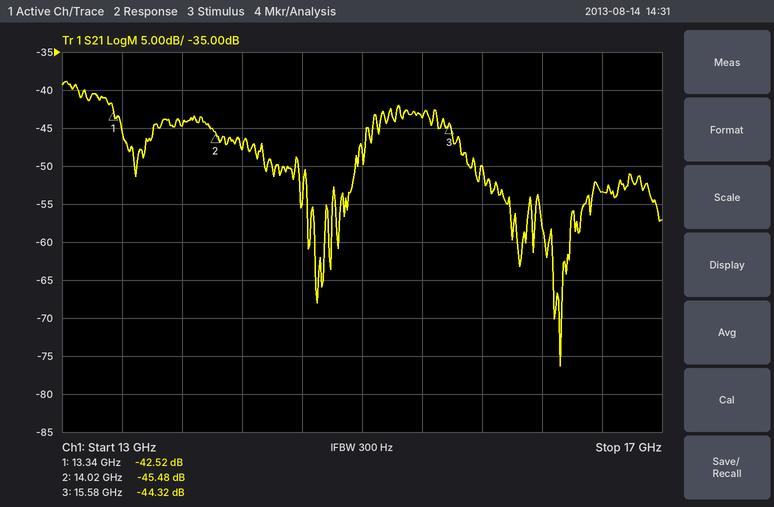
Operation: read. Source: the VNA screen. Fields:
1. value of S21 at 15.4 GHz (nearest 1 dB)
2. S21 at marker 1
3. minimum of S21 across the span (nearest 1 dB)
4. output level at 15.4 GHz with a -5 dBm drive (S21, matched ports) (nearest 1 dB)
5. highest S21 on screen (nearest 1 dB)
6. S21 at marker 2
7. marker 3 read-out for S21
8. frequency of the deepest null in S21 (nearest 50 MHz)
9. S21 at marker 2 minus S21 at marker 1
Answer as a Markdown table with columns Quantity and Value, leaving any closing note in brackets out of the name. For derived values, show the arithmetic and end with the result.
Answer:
| Quantity | Value |
|---|---|
| value of S21 at 15.4 GHz | -44 dB |
| S21 at marker 1 | -42.52 dB |
| minimum of S21 across the span | -76 dB |
| output level at 15.4 GHz with a -5 dBm drive (S21, matched ports) | -5 dBm + (-44 dB) = -49 dBm |
| highest S21 on screen | -39 dB |
| S21 at marker 2 | -45.48 dB |
| marker 3 read-out for S21 | -44.32 dB |
| frequency of the deepest null in S21 | 16.30 GHz |
| S21 at marker 2 minus S21 at marker 1 | -45.48 − (-42.52) = -2.96 dB |
